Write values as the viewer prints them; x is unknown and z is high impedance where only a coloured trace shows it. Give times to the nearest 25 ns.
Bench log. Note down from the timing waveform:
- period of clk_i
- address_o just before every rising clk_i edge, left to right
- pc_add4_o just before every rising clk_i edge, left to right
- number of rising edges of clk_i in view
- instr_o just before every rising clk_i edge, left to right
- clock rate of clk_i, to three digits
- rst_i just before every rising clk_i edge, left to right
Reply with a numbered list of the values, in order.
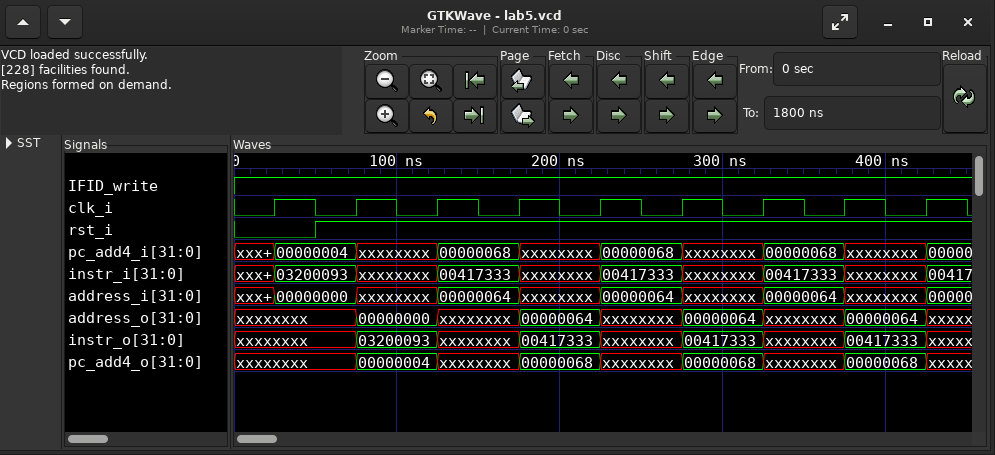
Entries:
1. 50 ns
2. xxxxxxxx, xxxxxxxx, 00000000, xxxxxxxx, 00000064, xxxxxxxx, 00000064, xxxxxxxx, 00000064
3. xxxxxxxx, xxxxxxxx, 00000004, xxxxxxxx, 00000068, xxxxxxxx, 00000068, xxxxxxxx, 00000068
4. 9
5. xxxxxxxx, xxxxxxxx, 03200093, xxxxxxxx, 00417333, xxxxxxxx, 00417333, xxxxxxxx, 00417333
6. 20.0 MHz
7. 0 1 1 1 1 1 1 1 1
